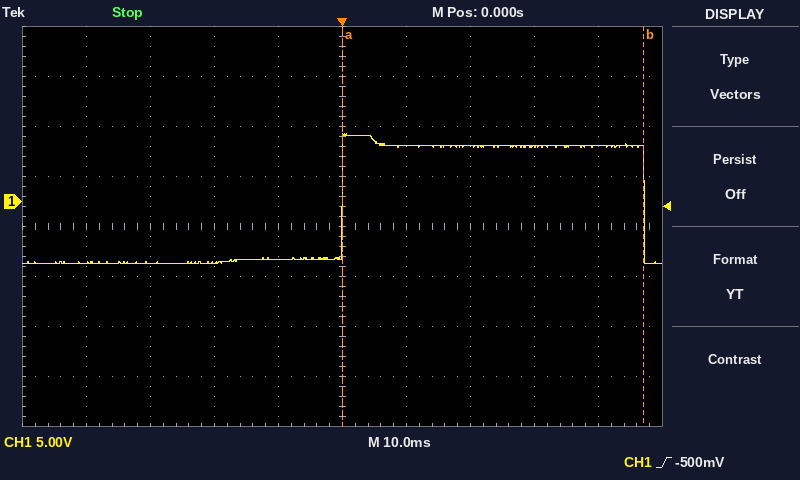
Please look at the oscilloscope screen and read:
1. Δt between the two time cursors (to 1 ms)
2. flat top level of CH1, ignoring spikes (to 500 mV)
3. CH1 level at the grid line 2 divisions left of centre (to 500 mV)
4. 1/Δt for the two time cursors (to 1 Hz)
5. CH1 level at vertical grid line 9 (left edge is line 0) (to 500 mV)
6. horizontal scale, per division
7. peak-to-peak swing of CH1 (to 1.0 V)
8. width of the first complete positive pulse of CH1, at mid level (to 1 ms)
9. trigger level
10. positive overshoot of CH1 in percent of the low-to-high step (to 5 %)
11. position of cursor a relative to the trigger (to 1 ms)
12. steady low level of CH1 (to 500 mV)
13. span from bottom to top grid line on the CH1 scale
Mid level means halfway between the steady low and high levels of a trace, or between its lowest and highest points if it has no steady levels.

47 ms
5.5 V
-6.0 V
21 Hz
5.5 V
10 ms
13.0 V
47 ms
-500 mV
10 %
0 ms
-6.0 V
40 V
